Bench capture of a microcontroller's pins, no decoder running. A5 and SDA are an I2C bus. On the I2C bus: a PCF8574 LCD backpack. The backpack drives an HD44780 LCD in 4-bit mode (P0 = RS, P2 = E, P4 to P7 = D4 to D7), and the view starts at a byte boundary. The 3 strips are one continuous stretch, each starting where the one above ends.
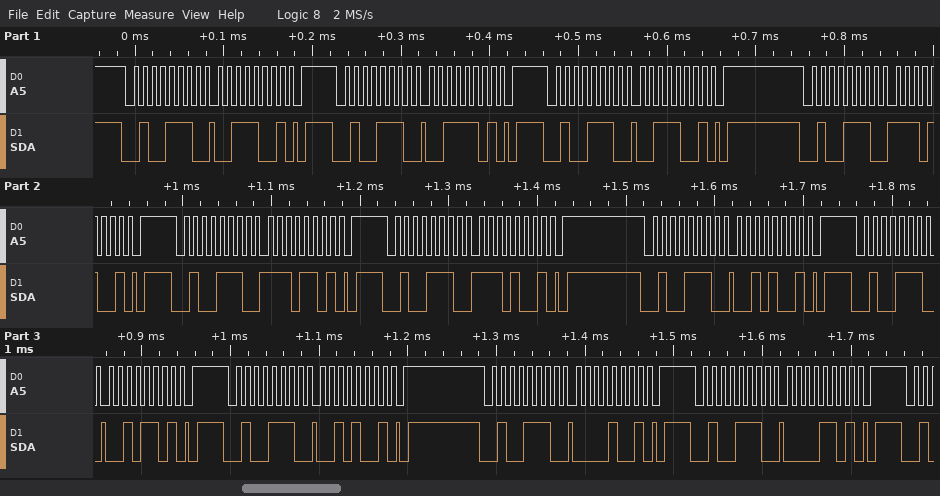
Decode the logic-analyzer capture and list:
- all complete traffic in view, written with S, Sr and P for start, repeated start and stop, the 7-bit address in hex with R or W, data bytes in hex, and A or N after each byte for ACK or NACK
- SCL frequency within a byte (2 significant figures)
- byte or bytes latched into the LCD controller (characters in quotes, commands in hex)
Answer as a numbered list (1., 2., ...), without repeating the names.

1. S 27W A 39 A P S 27W A 3D A P S 27W A 39 A P S 27W A E9 A P S 27W A ED A P S 27W A E9 A P S 27W A 29 A P S 27W A 2D A P S 27W A 29 A P S 27W A 09 A P S 27W A 0D A P
2. 100 kHz
3. '>'
